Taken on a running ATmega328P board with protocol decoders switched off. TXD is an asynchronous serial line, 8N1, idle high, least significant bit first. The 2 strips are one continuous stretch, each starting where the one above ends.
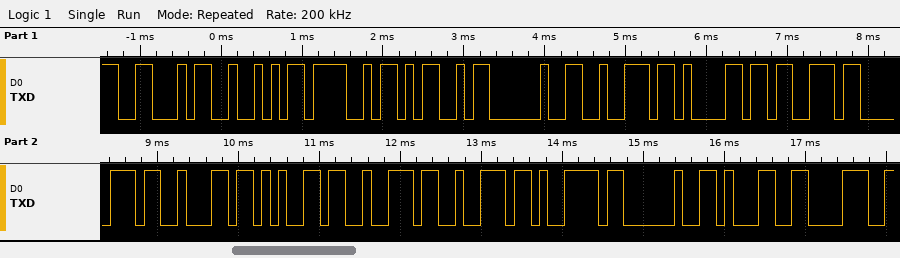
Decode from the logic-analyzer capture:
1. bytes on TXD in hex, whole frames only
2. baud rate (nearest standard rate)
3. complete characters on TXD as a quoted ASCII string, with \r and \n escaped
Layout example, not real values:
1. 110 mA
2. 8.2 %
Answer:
1. 46 52 4F 4D 20 72 61 73 70 62 65 72 72 79 20 31 38
2. 9600 baud
3. "FROM raspberry 18"
